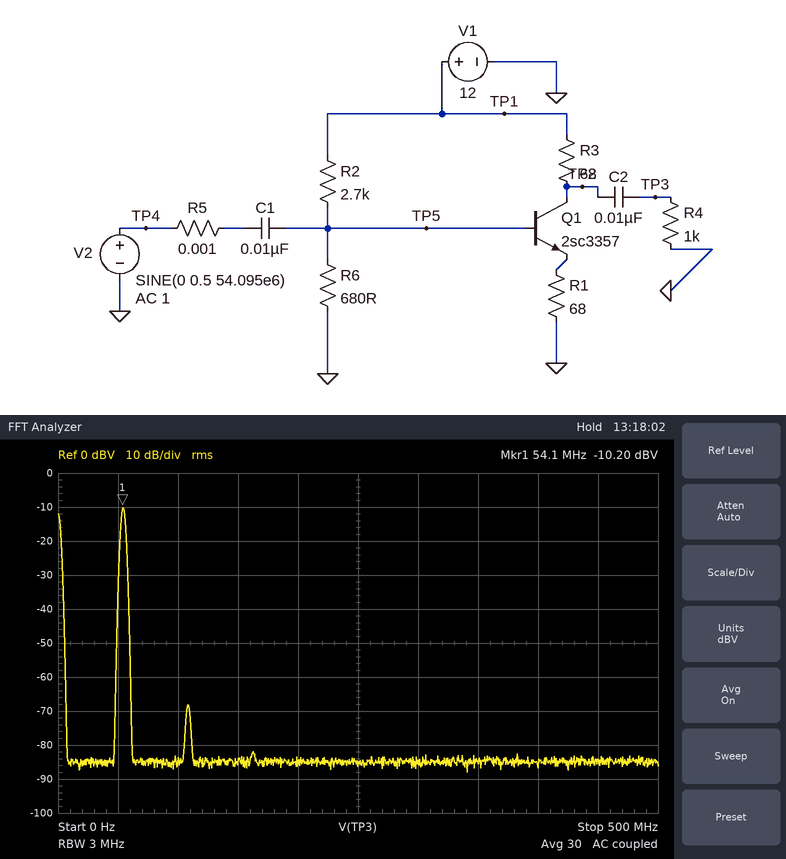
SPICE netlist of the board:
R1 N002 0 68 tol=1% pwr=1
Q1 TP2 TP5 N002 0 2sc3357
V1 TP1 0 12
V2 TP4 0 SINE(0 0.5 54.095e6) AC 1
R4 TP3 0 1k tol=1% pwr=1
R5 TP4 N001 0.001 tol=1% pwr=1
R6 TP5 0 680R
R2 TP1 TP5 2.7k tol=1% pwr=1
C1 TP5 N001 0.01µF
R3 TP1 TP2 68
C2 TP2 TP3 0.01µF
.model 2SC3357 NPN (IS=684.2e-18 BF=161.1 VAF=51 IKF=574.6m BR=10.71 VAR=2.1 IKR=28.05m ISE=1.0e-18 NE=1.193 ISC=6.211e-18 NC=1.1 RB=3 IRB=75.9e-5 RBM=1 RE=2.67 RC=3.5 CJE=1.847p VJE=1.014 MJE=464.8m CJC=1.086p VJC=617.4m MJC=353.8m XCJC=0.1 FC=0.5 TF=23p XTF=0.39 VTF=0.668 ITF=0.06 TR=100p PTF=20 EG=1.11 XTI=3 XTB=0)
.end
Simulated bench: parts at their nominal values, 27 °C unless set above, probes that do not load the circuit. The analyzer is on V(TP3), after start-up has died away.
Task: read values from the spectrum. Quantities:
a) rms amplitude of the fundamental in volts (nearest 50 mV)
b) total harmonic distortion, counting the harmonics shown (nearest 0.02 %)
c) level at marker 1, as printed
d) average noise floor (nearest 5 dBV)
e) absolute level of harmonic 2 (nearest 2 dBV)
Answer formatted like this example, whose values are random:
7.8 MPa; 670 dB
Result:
300 mV; 0.12 %; -10.20 dBV; -85 dBV; -68 dBV
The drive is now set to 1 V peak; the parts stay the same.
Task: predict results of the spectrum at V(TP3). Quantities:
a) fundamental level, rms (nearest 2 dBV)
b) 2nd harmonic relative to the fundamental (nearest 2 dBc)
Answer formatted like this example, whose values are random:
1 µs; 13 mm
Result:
-4 dBV; -50 dBc
